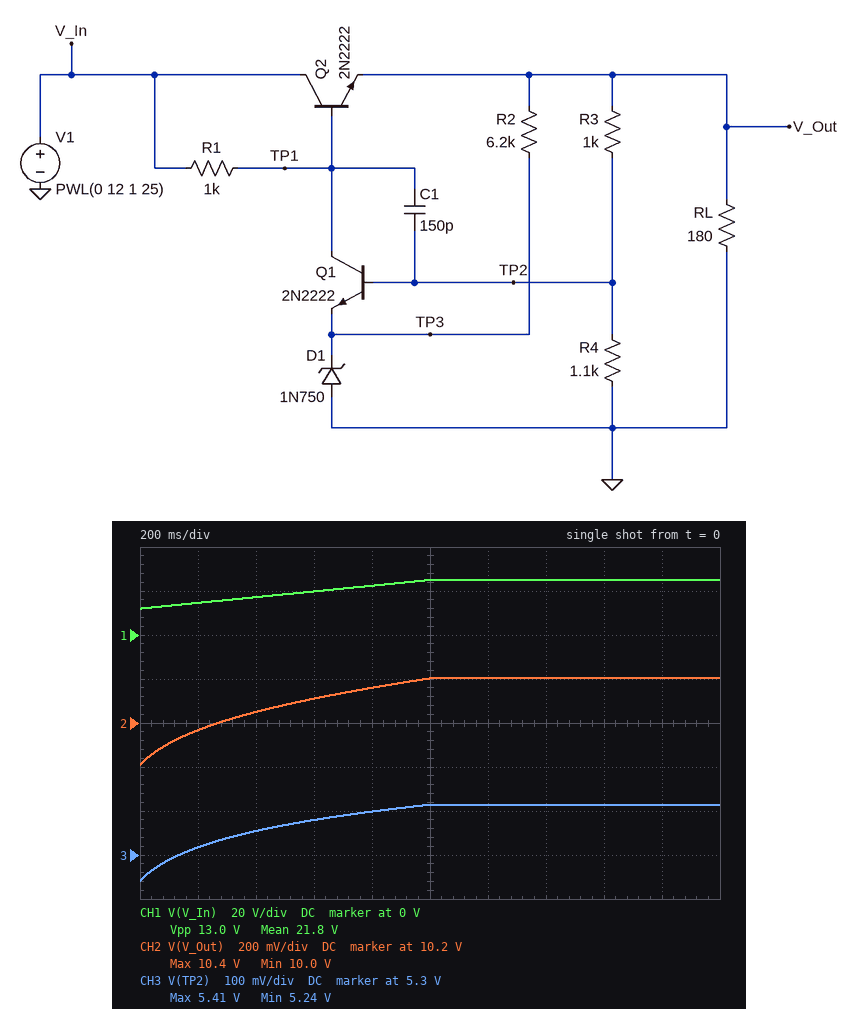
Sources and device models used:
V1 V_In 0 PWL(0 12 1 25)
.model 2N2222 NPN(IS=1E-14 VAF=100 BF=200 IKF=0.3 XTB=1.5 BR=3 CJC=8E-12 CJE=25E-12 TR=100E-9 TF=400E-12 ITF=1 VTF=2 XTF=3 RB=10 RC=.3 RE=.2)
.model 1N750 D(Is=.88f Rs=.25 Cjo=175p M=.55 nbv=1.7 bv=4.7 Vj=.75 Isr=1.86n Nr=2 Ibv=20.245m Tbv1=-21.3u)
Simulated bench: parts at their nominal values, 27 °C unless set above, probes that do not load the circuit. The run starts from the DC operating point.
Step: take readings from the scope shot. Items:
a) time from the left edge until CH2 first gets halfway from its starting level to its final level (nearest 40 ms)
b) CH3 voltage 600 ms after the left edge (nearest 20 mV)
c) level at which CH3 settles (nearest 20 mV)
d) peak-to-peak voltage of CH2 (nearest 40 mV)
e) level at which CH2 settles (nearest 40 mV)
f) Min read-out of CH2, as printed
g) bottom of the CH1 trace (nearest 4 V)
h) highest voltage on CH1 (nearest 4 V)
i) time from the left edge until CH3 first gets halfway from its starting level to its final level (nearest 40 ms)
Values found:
280 ms
5.38 V
5.42 V
400 mV
10.40 V
10.0 V
12 V
24 V
240 ms
